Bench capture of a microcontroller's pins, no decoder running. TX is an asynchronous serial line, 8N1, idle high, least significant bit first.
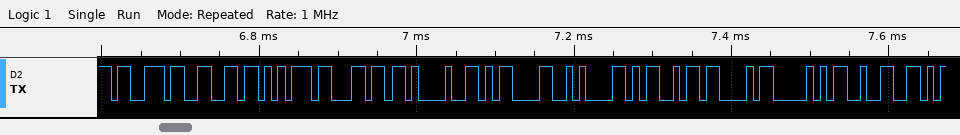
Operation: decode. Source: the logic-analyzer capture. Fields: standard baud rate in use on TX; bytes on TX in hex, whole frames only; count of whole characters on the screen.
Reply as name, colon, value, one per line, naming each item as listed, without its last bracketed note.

standard baud rate in use on TX: 115200 baud
bytes on TX in hex, whole frames only: 0x73 0x66 0x75 0x6C 0x21 0x0D 0x0A 0x4D 0x43 0x50 0x32
count of whole characters on the screen: 11
